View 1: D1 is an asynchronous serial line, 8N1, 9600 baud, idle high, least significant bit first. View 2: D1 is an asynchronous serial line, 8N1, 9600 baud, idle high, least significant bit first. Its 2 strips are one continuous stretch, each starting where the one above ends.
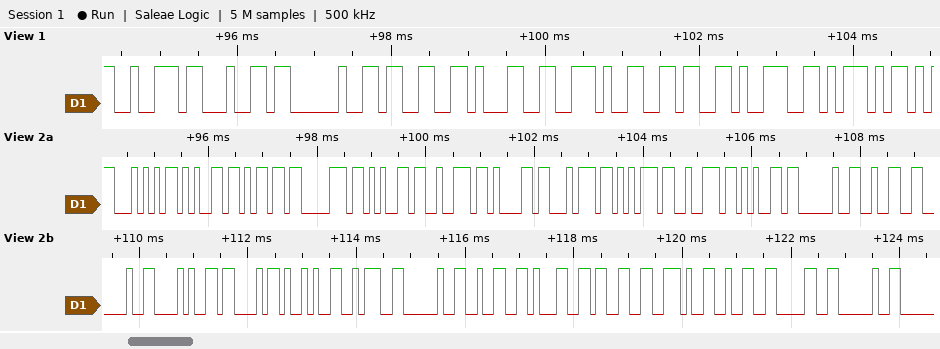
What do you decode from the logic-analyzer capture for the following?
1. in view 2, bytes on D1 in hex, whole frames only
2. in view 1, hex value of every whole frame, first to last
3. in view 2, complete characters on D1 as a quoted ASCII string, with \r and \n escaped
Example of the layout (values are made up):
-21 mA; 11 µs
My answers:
0x54 0x65 0x6D 0x70 0x65 0x72 0x61 0x74 0x75 0x72 0x65 0x20 0x32 0x20 0x28 0x43 0x29 0x3A 0x20 0x32 0x31 0x33 0x2E 0x32 0x30 0x20; 72 64 20 33 31 2E 36 39 5D; "Temperature 2 (C): 213.20 "
